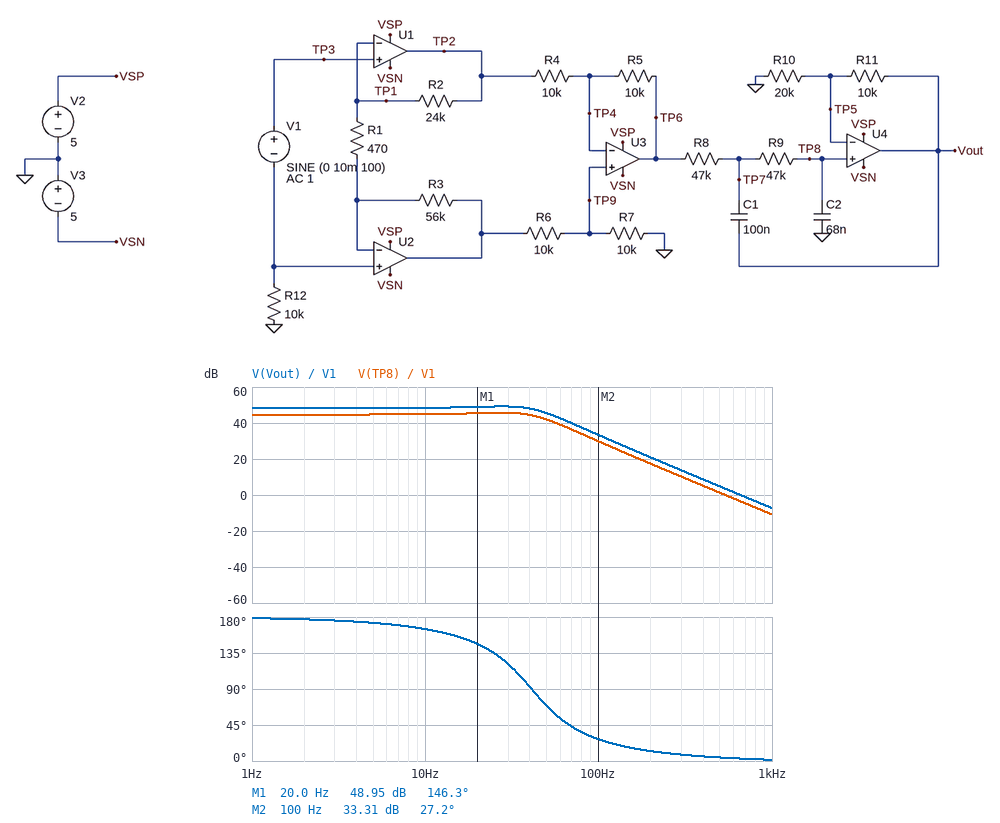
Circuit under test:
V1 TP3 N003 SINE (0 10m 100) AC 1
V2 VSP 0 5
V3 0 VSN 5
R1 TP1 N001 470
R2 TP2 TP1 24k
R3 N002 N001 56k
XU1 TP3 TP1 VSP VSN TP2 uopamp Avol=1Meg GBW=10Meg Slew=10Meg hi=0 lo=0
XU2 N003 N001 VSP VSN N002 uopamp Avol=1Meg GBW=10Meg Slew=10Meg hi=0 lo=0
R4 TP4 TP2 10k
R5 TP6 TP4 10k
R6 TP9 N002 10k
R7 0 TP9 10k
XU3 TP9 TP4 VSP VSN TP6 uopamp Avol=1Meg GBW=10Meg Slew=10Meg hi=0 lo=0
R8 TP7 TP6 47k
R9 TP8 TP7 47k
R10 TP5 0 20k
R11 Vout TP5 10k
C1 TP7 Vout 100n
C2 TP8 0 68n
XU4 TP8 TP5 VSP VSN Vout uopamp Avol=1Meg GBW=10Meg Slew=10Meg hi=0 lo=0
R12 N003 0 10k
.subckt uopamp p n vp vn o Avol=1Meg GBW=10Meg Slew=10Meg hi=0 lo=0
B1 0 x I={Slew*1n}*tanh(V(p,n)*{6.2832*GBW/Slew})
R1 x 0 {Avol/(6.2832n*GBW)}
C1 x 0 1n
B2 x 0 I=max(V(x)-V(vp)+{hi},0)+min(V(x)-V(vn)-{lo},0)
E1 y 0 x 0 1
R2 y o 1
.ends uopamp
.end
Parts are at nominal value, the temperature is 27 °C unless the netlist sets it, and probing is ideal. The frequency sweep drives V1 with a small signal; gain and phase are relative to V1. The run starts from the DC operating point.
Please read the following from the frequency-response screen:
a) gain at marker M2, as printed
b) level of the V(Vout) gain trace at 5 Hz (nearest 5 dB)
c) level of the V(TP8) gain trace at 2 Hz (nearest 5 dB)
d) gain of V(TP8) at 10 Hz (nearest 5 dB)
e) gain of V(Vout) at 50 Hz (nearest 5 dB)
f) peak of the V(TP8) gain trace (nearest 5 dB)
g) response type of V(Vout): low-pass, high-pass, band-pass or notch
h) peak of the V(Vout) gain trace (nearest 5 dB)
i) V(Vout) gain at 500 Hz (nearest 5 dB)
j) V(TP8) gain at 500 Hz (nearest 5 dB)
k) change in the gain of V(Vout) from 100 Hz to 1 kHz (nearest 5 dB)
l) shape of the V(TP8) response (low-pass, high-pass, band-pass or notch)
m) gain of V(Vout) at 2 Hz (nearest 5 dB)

33.31 dB
50 dB
45 dB
45 dB
45 dB
45 dB
low-pass
50 dB
5 dB
0 dB
-40 dB
low-pass
50 dB
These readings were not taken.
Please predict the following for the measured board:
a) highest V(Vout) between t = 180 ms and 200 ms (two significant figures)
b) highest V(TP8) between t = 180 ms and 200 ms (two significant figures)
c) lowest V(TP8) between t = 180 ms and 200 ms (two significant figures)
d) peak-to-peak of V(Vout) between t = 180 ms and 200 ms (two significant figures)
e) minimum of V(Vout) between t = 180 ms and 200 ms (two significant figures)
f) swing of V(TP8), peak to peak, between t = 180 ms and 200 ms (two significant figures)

460 mV
310 mV
-310 mV
930 mV
-460 mV
620 mV
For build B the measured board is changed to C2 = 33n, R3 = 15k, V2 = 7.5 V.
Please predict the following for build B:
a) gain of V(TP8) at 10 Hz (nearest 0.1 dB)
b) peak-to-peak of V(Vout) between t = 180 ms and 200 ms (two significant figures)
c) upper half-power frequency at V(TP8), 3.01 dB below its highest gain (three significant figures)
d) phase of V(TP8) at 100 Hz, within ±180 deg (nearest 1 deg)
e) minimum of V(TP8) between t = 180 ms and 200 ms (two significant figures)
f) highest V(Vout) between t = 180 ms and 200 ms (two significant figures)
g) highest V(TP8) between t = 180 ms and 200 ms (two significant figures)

38.7 dB
1.3 V
65.6 Hz
14 deg
-430 mV
650 mV
430 mV
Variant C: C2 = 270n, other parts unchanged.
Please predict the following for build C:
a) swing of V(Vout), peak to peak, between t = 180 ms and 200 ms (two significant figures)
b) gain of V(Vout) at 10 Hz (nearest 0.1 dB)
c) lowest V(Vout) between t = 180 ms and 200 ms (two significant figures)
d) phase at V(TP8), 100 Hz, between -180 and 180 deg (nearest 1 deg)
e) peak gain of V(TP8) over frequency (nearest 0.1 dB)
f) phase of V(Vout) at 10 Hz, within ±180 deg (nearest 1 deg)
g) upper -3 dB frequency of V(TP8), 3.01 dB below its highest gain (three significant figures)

190 mV
43.9 dB
-96 mV
33 deg
44.7 dB
118 deg
7.77 Hz
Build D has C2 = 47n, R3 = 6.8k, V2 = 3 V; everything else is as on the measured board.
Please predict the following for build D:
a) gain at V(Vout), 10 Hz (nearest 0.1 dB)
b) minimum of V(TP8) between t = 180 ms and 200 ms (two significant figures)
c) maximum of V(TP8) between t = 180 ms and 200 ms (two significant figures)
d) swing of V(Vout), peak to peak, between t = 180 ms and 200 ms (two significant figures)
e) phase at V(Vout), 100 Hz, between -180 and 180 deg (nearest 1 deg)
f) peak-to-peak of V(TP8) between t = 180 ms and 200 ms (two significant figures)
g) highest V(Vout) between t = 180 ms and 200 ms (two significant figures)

40.3 dB
-200 mV
200 mV
590 mV
23 deg
400 mV
300 mV
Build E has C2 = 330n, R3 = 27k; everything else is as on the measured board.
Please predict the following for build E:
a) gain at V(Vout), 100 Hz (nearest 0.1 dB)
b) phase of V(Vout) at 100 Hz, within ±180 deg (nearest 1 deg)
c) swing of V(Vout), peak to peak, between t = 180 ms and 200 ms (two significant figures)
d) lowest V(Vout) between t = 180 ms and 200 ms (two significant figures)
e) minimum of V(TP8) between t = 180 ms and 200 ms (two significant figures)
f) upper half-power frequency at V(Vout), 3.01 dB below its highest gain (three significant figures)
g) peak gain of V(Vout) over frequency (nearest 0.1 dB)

13.9 dB
33 deg
99 mV
-50 mV
-33 mV
6.09 Hz
44.3 dB
